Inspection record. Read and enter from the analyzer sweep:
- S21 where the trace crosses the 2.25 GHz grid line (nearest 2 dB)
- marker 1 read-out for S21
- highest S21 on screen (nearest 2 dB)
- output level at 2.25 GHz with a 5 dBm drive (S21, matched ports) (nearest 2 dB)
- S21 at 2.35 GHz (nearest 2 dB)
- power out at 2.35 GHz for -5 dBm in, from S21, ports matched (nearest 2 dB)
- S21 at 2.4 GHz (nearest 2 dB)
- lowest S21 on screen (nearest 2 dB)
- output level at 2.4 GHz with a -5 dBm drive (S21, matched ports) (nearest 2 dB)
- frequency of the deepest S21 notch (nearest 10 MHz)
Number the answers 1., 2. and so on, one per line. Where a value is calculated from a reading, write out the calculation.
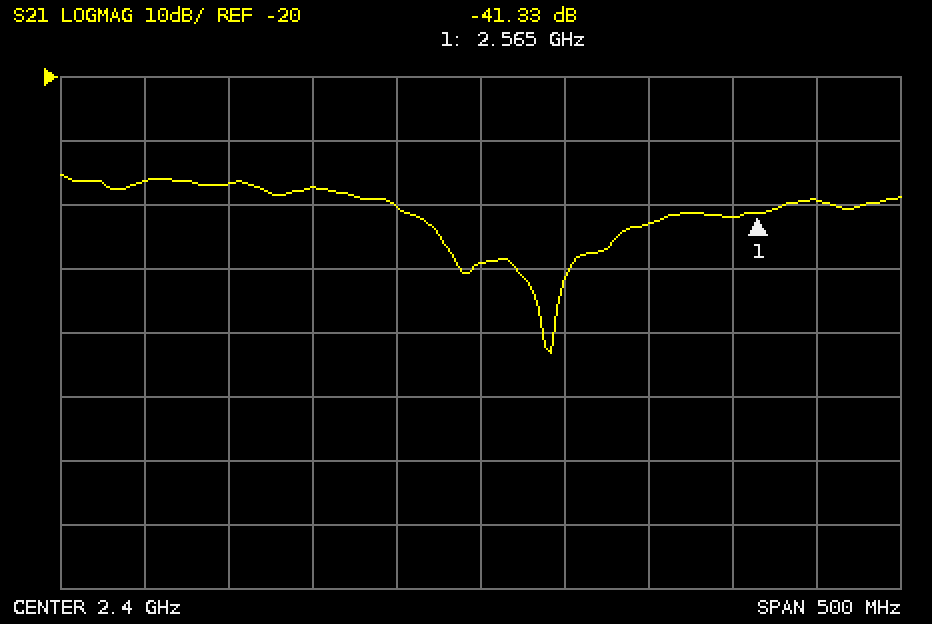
1. -36 dB
2. -41.33 dB
3. -36 dB
4. 5 dBm + (-36 dB) = -32 dBm
5. -40 dB
6. -5 dBm + (-40 dB) = -46 dBm
7. -50 dB
8. -64 dB
9. -5 dBm + (-50 dB) = -54 dBm
10. 2.44 GHz
